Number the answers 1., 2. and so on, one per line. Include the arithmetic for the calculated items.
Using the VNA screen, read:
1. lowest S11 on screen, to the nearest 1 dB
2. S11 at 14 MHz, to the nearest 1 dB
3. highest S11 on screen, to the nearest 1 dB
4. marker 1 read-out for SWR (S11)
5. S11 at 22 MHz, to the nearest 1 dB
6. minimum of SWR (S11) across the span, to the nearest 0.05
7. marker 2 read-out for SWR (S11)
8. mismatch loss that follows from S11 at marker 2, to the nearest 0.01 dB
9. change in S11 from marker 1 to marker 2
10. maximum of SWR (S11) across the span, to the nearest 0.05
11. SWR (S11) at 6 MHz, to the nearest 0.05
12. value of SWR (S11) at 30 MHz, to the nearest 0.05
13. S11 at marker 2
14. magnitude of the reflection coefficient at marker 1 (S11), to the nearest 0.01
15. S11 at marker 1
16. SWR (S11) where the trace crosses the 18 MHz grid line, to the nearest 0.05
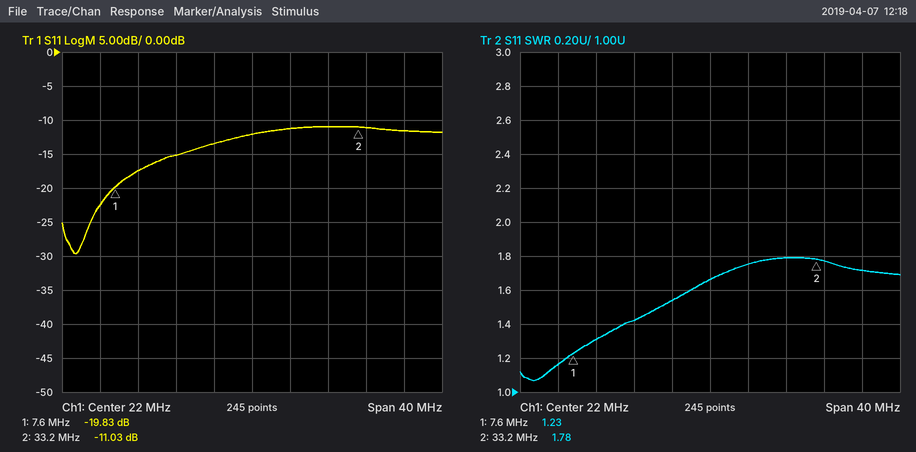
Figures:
1. -30 dB
2. -15 dB
3. -11 dB
4. 1.23
5. -12 dB
6. 1.05
7. 1.78
8. −10 log10(1 − 10^(-11.03/10)) ≈ 0.36 dB
9. -11.03 − (-19.83) = 8.80 dB
10. 1.80
11. 1.15
12. 1.80
13. -11.03 dB
14. 10^(-19.83/20) ≈ 0.10
15. -19.83 dB
16. 1.55
